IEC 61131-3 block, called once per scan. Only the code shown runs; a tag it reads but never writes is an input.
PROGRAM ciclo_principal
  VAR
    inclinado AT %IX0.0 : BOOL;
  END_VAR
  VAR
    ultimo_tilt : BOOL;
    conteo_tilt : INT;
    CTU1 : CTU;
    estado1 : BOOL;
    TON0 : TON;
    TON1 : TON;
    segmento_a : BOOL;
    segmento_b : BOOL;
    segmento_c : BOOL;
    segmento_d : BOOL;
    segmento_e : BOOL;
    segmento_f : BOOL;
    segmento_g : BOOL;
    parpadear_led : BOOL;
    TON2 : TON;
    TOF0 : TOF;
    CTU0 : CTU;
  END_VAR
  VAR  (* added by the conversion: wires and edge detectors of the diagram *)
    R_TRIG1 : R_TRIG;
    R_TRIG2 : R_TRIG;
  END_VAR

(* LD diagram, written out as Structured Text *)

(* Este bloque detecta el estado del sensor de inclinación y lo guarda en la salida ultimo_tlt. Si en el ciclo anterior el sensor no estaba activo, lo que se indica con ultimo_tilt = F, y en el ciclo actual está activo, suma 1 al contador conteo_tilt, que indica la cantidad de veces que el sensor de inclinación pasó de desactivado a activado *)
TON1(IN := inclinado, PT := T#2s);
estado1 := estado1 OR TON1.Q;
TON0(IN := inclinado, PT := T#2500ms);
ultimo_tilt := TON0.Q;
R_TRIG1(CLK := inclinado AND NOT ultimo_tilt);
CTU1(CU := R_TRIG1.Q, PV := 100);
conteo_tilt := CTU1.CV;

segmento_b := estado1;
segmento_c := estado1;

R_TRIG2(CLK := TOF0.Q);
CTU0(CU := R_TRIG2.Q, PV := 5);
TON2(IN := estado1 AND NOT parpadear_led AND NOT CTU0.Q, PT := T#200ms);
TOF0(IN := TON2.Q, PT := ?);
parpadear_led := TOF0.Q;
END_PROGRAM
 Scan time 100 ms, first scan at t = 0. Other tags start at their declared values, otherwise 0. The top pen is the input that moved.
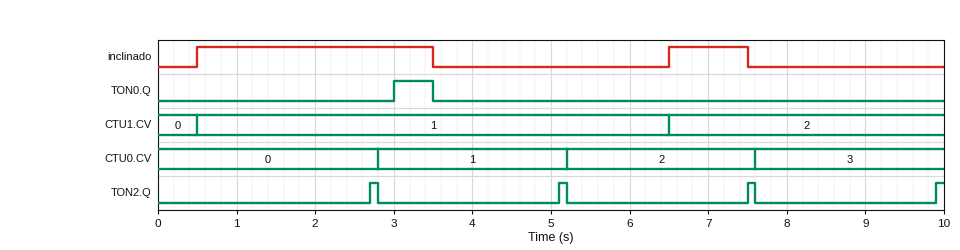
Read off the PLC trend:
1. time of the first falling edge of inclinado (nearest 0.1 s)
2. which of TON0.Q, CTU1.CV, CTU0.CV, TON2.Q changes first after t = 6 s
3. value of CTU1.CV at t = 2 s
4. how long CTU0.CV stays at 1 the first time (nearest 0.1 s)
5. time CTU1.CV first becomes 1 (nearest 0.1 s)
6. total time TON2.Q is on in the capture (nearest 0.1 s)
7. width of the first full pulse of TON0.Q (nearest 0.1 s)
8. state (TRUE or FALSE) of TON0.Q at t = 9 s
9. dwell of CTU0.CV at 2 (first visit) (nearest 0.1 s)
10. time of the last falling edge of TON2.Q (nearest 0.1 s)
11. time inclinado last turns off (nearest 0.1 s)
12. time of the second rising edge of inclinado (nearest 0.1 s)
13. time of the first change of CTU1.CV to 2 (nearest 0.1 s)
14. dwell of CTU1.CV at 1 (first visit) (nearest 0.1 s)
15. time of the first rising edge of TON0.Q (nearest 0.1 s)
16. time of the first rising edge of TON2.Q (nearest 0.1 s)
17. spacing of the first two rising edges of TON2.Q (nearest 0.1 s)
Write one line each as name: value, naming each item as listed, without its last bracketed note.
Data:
time of the first falling edge of inclinado: 3.5 s
which of TON0.Q, CTU1.CV, CTU0.CV, TON2.Q changes first after t = 6 s: CTU1.CV
value of CTU1.CV at t = 2 s: 1
how long CTU0.CV stays at 1 the first time: 2.4 s
time CTU1.CV first becomes 1: 0.5 s
total time TON2.Q is on in the capture: 0.4 s
width of the first full pulse of TON0.Q: 0.5 s
state (TRUE or FALSE) of TON0.Q at t = 9 s: FALSE
dwell of CTU0.CV at 2 (first visit): 2.4 s
time of the last falling edge of TON2.Q: 7.6 s
time inclinado last turns off: 7.5 s
time of the second rising edge of inclinado: 6.5 s
time of the first change of CTU1.CV to 2: 6.5 s
dwell of CTU1.CV at 1 (first visit): 6.0 s
time of the first rising edge of TON0.Q: 3.0 s
time of the first rising edge of TON2.Q: 2.7 s
spacing of the first two rising edges of TON2.Q: 2.4 s
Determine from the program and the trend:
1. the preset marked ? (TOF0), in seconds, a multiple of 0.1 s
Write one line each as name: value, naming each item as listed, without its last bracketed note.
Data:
the preset marked ? (TOF0), in seconds, a multiple of 0.1 s: 2.0 s
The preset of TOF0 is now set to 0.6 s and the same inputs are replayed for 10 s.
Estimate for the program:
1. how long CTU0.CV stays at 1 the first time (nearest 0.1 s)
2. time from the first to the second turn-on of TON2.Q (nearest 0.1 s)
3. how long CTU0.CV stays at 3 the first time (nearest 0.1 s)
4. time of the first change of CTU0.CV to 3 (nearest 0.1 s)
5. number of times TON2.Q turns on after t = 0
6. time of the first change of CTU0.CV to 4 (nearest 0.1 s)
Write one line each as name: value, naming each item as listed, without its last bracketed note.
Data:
how long CTU0.CV stays at 1 the first time: 1.0 s
time from the first to the second turn-on of TON2.Q: 1.0 s
how long CTU0.CV stays at 3 the first time: 1.0 s
time of the first change of CTU0.CV to 3: 4.8 s
number of times TON2.Q turns on after t = 0: 5
time of the first change of CTU0.CV to 4: 5.8 s
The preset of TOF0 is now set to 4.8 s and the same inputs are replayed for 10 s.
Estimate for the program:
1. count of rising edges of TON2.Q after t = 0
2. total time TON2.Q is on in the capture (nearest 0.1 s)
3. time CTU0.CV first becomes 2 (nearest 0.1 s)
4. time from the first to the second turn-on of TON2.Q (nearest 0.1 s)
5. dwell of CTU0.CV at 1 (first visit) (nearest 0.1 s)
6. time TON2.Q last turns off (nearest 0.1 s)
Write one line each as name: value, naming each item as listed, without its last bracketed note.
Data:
count of rising edges of TON2.Q after t = 0: 2
total time TON2.Q is on in the capture: 0.2 s
time CTU0.CV first becomes 2: 8.0 s
time from the first to the second turn-on of TON2.Q: 5.2 s
dwell of CTU0.CV at 1 (first visit): 5.2 s
time TON2.Q last turns off: 8.0 s
